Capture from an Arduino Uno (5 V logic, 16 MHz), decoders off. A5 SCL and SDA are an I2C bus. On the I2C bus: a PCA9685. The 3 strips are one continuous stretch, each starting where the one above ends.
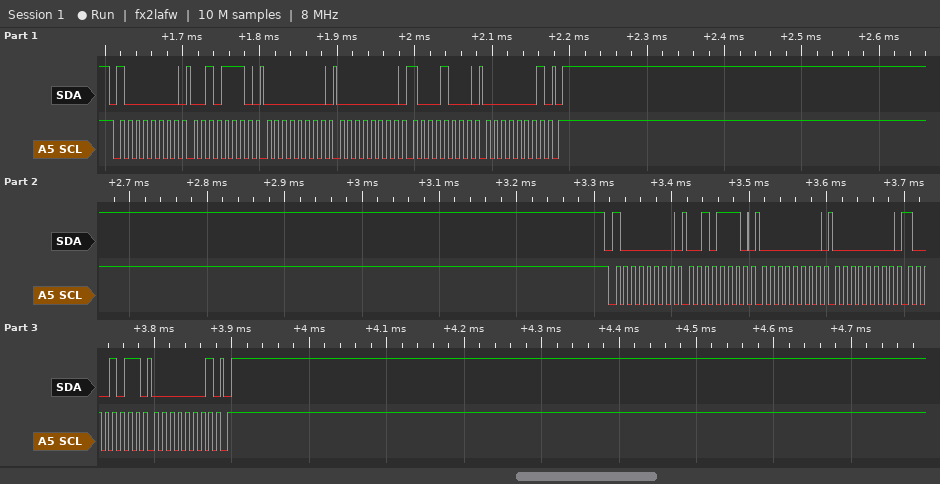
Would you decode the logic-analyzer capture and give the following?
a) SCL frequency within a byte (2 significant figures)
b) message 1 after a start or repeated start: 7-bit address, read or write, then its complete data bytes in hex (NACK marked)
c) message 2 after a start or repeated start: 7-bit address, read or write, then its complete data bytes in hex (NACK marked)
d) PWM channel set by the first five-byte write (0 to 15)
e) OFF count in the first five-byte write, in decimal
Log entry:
100 kHz
0x40 write: 2E 00 00 88 01
0x40 write: 2E 00 00 8B 01
10
392
